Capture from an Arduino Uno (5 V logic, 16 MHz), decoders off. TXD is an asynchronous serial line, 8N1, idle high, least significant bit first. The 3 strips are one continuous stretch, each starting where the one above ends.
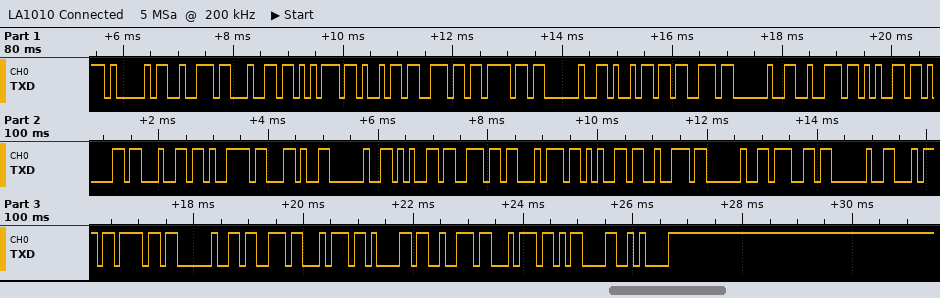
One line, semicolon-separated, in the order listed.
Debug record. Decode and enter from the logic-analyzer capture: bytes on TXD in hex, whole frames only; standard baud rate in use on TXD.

0x41 0x72 0x64 0x75 0x69 0x6E 0x6F 0x20 0x69 0x73 0x20 0x72 0x65 0x61 0x64 0x79 0x2C 0x20 0x65 0x6E 0x74 0x65 0x72 0x20 0x67 0x20 0x74 0x6F 0x20 0x73 0x74 0x61 0x72 0x74 0x0D 0x0A; 9600 baud
